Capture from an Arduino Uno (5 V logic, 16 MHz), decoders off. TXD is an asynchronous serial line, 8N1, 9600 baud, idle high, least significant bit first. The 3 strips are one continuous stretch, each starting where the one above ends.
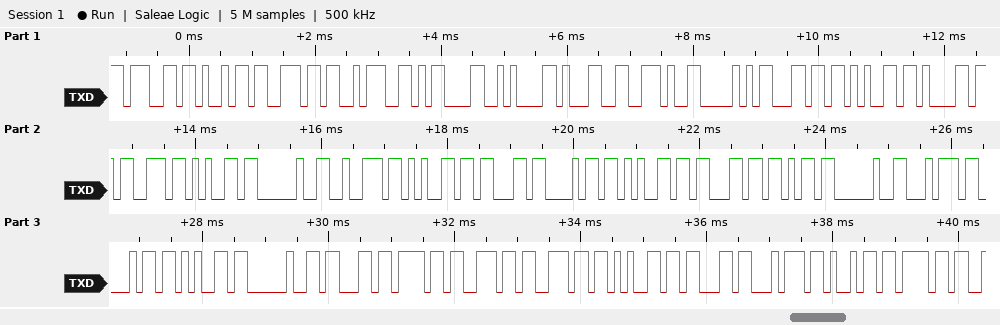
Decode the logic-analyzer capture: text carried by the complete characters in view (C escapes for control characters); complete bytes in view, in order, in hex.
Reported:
"gin:\r\n1.Please recheck the connectio"
67 69 6E 3A 0D 0A 31 2E 50 6C 65 61 73 65 20 72 65 63 68 65 63 6B 20 74 68 65 20 63 6F 6E 6E 65 63 74 69 6F
